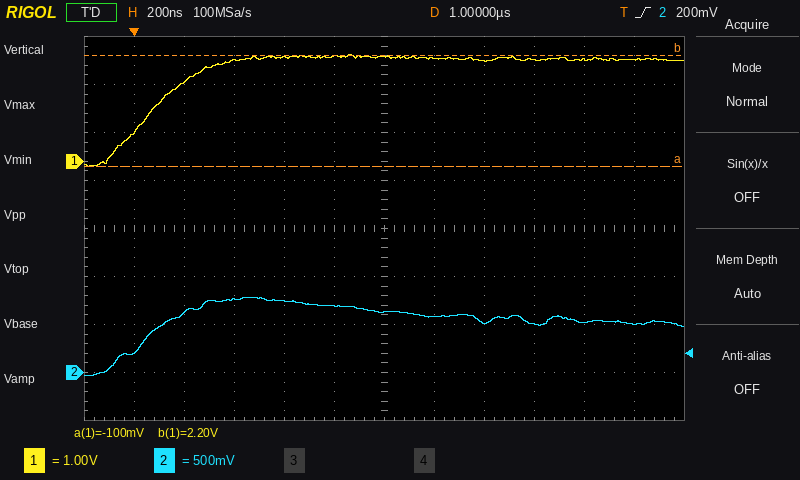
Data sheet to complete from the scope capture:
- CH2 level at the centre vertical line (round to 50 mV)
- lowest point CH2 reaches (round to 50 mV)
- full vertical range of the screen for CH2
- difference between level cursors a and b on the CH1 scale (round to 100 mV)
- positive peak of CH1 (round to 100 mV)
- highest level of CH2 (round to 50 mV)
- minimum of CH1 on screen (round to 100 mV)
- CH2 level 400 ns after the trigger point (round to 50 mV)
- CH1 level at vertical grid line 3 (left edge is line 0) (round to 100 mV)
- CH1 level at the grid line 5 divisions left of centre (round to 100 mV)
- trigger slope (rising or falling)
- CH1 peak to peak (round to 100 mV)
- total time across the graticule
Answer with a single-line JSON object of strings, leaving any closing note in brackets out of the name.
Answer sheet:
{"CH2 level at the centre vertical line": "650 mV", "lowest point CH2 reaches": "-50 mV", "full vertical range of the screen for CH2": "4 V", "difference between level cursors a and b on the CH1 scale": "2.3 V", "positive peak of CH1": "2.2 V", "highest level of CH2": "800 mV", "minimum of CH1 on screen": "-100 mV", "CH2 level 400 ns after the trigger point": "750 mV", "CH1 level at vertical grid line 3 (left edge is line 0)": "2.1 V", "CH1 level at the grid line 5 divisions left of centre": "600 mV", "trigger slope": "rising", "CH1 peak to peak": "2.3 V", "total time across the graticule": "2.4 µs"}
